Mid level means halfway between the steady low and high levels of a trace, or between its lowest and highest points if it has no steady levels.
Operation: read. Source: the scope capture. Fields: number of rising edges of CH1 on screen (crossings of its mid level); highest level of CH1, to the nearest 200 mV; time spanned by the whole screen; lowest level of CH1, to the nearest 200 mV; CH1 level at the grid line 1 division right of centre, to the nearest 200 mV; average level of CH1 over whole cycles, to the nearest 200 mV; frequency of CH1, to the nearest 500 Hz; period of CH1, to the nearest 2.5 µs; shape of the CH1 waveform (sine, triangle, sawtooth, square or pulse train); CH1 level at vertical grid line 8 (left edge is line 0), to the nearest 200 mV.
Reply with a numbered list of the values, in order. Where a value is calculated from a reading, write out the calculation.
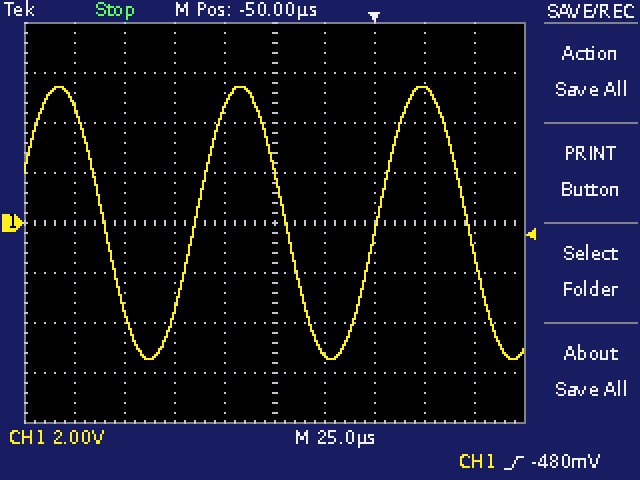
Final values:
1. 2
2. 5.4 V
3. 250 µs
4. -5.4 V
5. -5.2 V
6. (5.4 V + (-5.4 V)) / 2 ≈ 0.0 V
7. 1 / 90.0 µs ≈ 11.1 kHz, so 11.0 kHz to the nearest 500 Hz
8. 90.0 µs
9. sine
10. 5.4 V
